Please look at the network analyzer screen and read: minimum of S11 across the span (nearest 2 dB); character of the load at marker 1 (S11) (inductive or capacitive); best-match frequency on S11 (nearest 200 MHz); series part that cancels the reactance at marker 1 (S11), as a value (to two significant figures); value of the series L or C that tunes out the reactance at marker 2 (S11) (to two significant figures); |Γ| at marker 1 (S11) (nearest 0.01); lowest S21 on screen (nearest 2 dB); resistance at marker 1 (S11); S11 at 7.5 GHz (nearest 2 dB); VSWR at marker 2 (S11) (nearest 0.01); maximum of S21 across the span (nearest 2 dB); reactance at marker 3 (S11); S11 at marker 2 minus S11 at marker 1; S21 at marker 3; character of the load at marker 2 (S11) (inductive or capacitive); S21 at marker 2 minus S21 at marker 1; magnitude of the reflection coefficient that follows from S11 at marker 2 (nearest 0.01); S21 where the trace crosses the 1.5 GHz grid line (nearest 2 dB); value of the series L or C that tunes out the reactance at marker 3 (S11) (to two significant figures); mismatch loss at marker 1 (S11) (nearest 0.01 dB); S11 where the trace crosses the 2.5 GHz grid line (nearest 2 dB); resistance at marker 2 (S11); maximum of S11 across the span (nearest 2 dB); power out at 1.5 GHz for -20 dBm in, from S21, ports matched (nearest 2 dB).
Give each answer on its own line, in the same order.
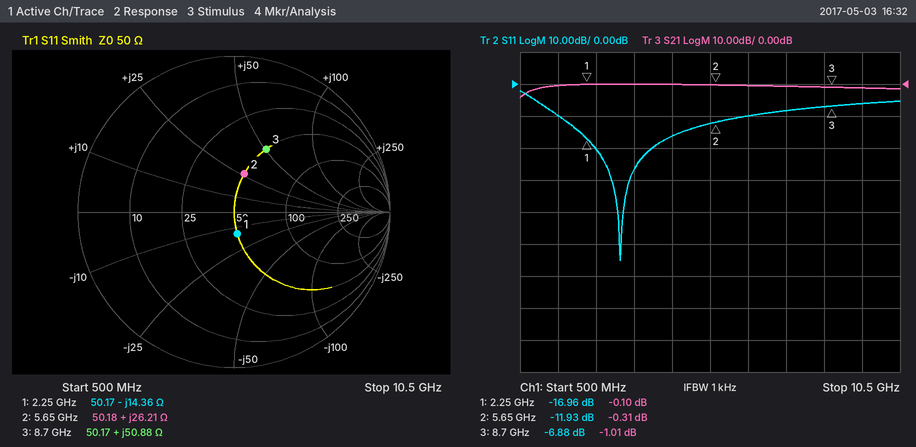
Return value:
-56 dB
capacitive
3.2 GHz
1.0 nH
1.1 pF
0.14
-4 dB
50.17 Ω
-8 dB
1.68
0 dB
+50.88 Ω
5.03 dB
-1.01 dB
inductive
-0.21 dB
0.25
0 dB
360 fF
0.09 dB
-20 dB
50.18 Ω
-2 dB
-20 dBm
